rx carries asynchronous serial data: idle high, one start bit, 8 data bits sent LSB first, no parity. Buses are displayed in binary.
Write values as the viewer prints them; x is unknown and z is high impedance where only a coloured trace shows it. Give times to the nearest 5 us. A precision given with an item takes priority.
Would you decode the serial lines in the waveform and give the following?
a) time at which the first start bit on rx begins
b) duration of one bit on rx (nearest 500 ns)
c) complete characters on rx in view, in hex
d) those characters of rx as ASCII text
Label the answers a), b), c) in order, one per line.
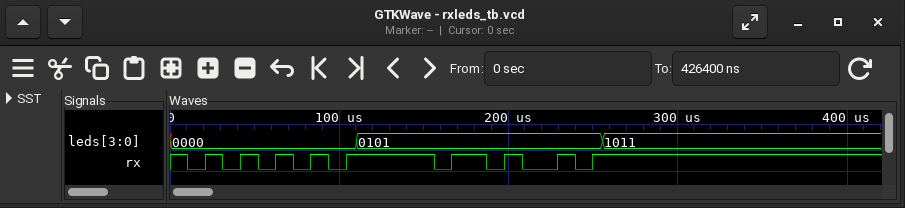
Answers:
a) 10 us
b) 10500 ns
c) 55, 4B
d) "UK"
